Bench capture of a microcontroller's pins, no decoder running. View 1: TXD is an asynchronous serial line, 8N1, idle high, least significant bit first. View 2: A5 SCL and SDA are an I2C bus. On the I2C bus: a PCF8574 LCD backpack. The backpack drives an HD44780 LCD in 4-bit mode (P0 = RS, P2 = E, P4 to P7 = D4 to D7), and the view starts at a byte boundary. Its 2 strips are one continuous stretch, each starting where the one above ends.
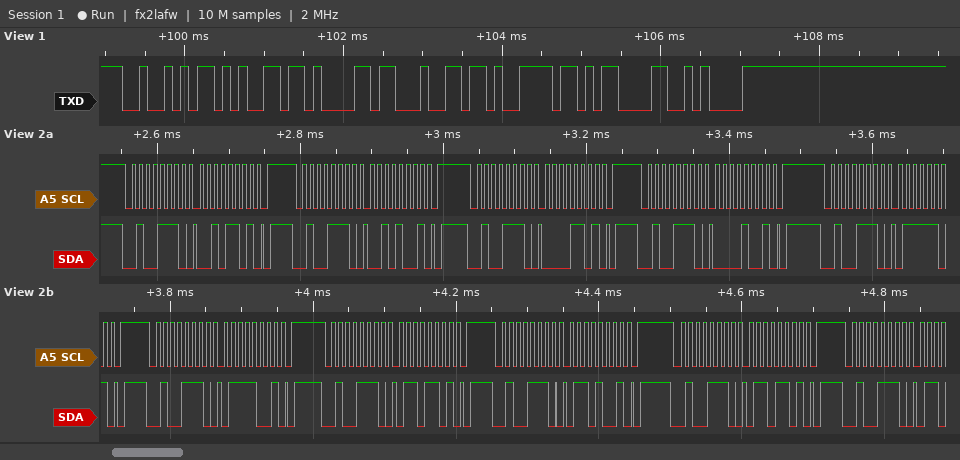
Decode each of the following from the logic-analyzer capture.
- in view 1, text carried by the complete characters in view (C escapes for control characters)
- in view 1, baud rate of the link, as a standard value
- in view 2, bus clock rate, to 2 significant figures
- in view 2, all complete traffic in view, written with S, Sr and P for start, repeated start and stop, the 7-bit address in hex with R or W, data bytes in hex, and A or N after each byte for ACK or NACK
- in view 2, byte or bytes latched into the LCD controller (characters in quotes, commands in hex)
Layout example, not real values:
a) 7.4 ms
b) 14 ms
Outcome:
a) "Ready\r\n"
b) 9600 baud
c) 100 kHz
d) S 27W A 2D A P S 27W A 29 A P S 27W A 0D A P S 27W A 09 A P S 27W A 7D A P S 27W A 79 A P S 27W A 6D A P S 27W A 69 A P S 27W A 6D A P S 27W A
e) ' ' 'v'
